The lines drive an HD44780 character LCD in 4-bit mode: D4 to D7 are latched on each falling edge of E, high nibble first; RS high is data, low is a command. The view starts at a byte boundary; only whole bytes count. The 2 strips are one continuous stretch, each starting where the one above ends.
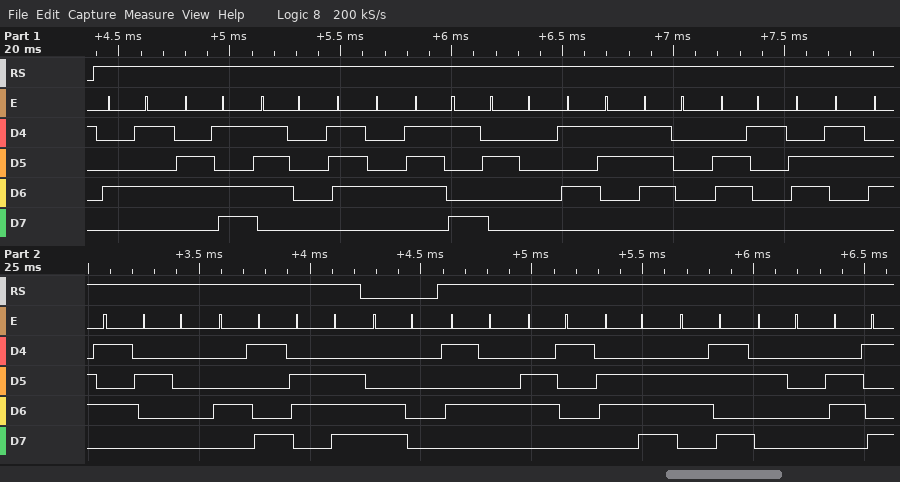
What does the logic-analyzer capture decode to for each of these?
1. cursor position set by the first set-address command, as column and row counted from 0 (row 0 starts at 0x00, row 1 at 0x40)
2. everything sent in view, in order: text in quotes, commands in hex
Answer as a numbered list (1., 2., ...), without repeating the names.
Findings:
1. column 0, row 1
2. "Empty Space In" 0xC0 "Tank i"
